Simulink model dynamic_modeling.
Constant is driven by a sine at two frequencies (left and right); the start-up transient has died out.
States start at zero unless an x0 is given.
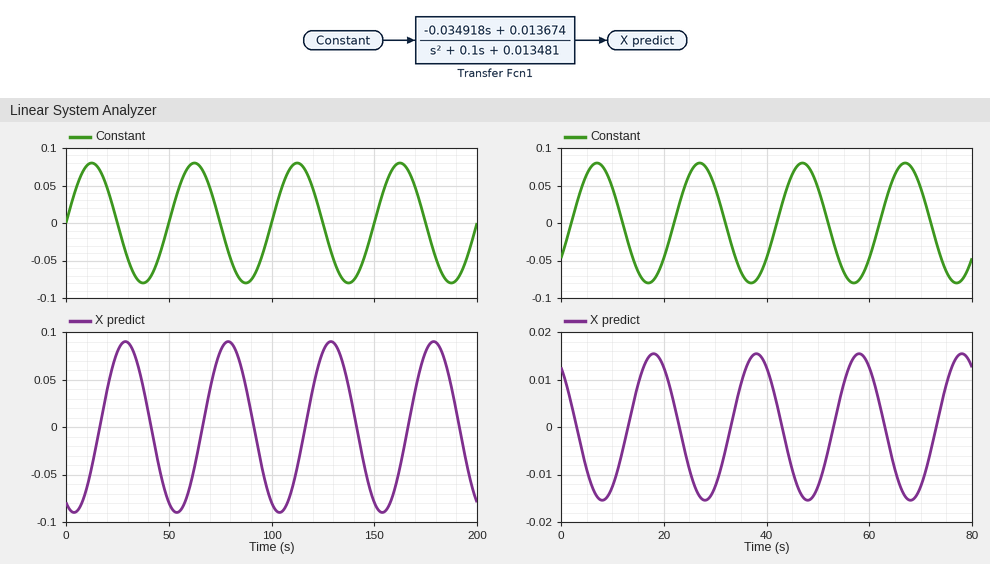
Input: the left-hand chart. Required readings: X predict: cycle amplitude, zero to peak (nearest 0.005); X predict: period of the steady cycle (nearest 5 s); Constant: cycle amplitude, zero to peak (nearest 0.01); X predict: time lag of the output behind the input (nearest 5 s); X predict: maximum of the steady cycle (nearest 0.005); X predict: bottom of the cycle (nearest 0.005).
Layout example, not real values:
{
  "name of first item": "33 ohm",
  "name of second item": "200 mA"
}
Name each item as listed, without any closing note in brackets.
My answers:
{
  "X predict: cycle amplitude, zero to peak": "0.090",
  "X predict: period of the steady cycle": "50 s",
  "Constant: cycle amplitude, zero to peak": "0.08",
  "X predict: time lag of the output behind the input": "15 s",
  "X predict: maximum of the steady cycle": "0.090",
  "X predict: bottom of the cycle": "-0.090"
}
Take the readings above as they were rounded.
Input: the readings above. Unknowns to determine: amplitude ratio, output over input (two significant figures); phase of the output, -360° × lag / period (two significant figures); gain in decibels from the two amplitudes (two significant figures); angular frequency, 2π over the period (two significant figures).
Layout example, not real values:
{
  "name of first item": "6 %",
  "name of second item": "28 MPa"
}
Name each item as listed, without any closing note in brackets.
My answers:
{
  "amplitude ratio, output over input": "1.1",
  "phase of the output, -360° × lag / period": "-110°",
  "gain in decibels from the two amplitudes": "1.0 dB",
  "angular frequency, 2π over the period": "0.13 rad/s"
}
